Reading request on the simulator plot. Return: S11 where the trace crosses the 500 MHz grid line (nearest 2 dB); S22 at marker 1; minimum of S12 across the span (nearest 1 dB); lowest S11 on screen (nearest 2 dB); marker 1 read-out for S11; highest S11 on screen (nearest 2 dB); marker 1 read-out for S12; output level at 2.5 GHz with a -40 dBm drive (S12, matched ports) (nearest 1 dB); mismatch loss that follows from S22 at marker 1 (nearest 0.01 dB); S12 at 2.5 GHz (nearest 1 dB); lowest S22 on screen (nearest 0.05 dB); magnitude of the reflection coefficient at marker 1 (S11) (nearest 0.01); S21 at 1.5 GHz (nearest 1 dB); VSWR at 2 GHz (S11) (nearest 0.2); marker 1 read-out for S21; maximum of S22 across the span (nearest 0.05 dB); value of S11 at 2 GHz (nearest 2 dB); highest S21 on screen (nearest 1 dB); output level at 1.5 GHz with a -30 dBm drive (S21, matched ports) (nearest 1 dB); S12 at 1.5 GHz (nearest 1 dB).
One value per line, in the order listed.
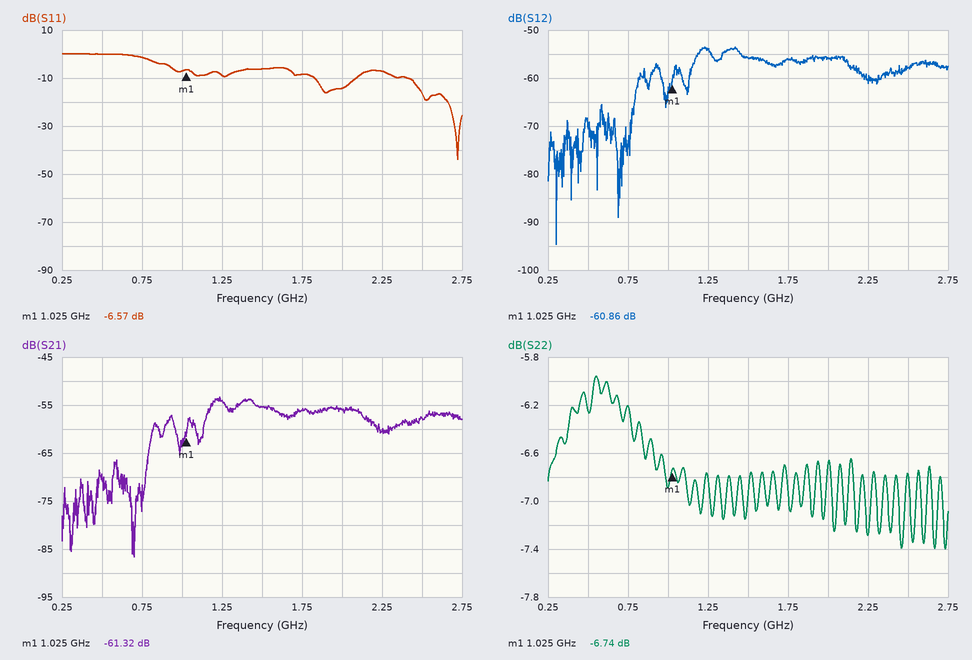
0 dB
-6.74 dB
-95 dB
-44 dB
-6.57 dB
0 dB
-60.86 dB
-98 dBm
1.03 dB
-58 dB
-7.40 dB
0.47
-55 dB
1.4
-61.32 dB
-5.95 dB
-14 dB
-53 dB
-85 dBm
-56 dB
